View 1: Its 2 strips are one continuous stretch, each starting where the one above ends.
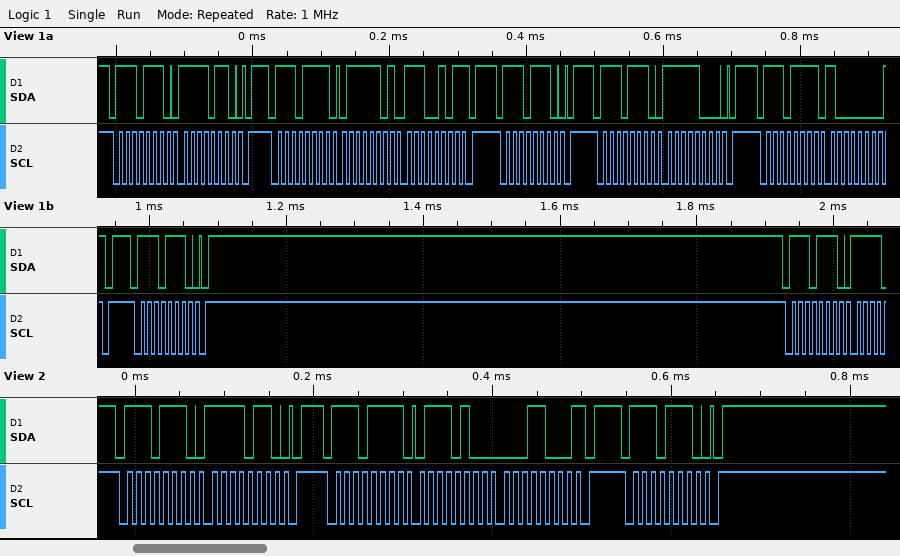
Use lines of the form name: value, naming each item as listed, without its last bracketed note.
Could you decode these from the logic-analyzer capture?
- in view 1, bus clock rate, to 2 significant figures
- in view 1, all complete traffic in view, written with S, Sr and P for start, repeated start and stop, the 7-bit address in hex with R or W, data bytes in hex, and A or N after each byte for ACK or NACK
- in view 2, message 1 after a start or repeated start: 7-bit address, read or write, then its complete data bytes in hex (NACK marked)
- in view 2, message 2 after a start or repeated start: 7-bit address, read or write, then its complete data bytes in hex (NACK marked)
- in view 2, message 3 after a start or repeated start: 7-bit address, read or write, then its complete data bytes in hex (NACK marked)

in view 1, bus clock rate, to 2 significant figures: 100 kHz
in view 1, all complete traffic in view, written with S, Sr and P for start, repeated start and stop, the 7-bit address in hex with R or W, data bytes in hex, and A or N after each byte for ACK or NACK: S 77W A F6 A P S 77R A 7D A E5 N P S 77W A P S 77W A F8 A P S 77R A 80 N P S 77W A P S 77W A
in view 2, message 1 after a start or repeated start: 7-bit address, read or write, then its complete data bytes in hex: 0x77 write: F6
in view 2, message 2 after a start or repeated start: 7-bit address, read or write, then its complete data bytes in hex: 0x77 read: 74 18 NACK
in view 2, message 3 after a start or repeated start: 7-bit address, read or write, then its complete data bytes in hex: 0x77 write
